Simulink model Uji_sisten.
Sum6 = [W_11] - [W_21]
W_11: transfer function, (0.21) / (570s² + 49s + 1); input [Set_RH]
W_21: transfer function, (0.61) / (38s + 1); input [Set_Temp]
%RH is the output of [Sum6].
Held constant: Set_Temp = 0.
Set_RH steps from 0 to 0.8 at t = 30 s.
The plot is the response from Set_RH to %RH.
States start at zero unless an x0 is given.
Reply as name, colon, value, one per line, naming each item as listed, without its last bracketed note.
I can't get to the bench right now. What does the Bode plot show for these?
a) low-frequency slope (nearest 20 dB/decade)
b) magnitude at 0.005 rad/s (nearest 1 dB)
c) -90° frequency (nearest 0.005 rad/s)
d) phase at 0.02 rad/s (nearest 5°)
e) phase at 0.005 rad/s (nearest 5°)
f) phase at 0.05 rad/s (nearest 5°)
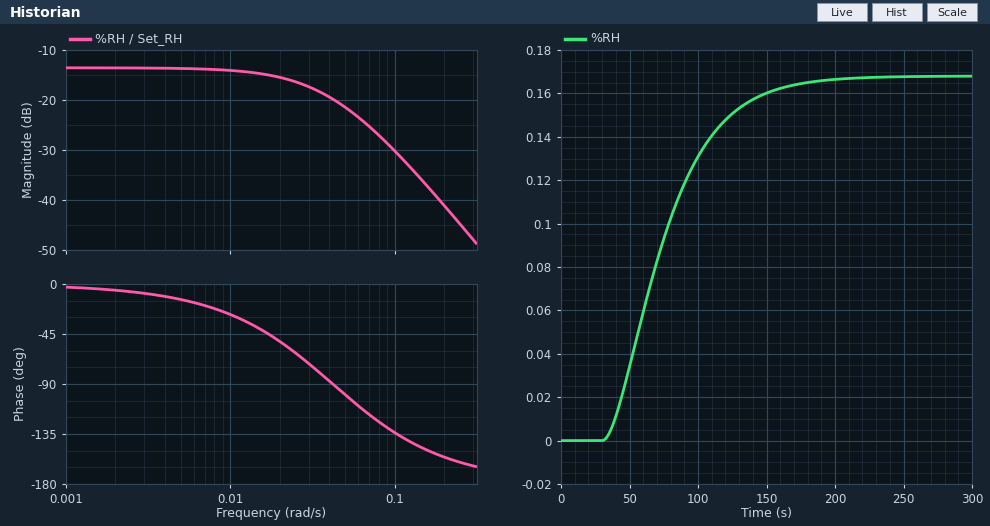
low-frequency slope: 0 dB/decade
magnitude at 0.005 rad/s: -14 dB
-90° frequency: 0.040 rad/s
phase at 0.02 rad/s: -50°
phase at 0.005 rad/s: -15°
phase at 0.05 rad/s: -100°
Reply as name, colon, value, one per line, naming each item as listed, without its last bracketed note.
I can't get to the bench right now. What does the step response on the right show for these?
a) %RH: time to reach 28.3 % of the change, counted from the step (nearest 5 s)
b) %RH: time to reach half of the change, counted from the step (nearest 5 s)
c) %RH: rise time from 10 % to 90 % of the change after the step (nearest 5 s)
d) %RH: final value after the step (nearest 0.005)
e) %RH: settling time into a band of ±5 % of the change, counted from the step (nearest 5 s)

%RH: time to reach 28.3 % of the change, counted from the step: 25 s
%RH: time to reach half of the change, counted from the step: 40 s
%RH: rise time from 10 % to 90 % of the change after the step: 85 s
%RH: final value after the step: 0.170
%RH: settling time into a band of ±5 % of the change, counted from the step: 120 s
